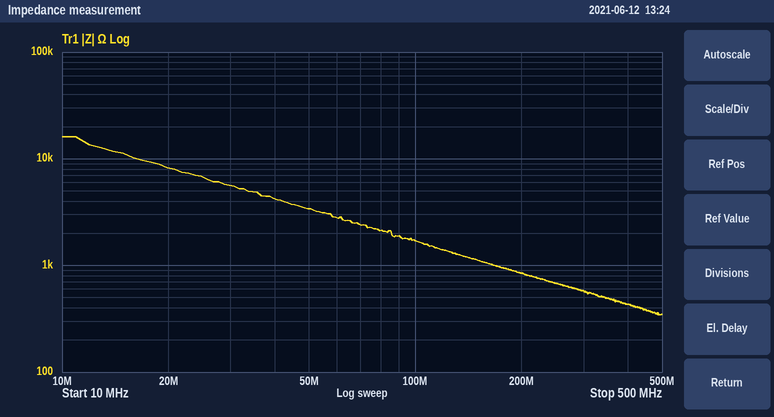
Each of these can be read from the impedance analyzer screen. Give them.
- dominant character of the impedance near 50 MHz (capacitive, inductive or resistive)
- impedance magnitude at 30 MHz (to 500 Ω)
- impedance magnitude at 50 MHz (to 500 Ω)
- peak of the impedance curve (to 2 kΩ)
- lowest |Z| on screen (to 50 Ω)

capacitive
5.5 kΩ
3.5 kΩ
16 kΩ
350 Ω
